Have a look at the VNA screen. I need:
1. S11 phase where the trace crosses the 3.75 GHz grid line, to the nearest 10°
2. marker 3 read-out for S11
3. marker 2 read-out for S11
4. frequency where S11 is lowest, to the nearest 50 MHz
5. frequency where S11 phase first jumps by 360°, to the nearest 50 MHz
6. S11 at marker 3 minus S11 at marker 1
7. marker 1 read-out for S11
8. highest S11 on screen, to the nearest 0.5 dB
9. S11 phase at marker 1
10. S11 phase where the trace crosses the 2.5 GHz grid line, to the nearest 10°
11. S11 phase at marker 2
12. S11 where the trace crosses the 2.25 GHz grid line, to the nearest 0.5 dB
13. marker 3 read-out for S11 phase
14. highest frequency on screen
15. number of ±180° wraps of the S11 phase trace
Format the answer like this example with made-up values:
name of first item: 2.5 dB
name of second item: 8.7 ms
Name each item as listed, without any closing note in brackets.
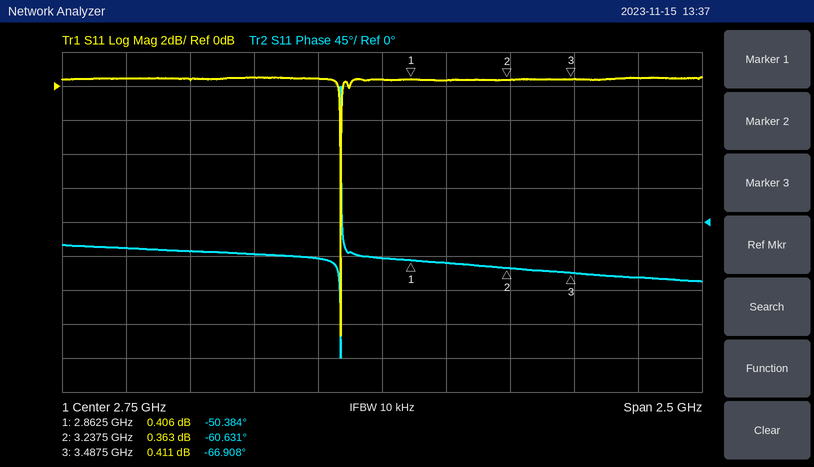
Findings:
S11 phase where the trace crosses the 3.75 GHz grid line, to the nearest 10°: -70°
marker 3 read-out for S11: 0.411 dB
marker 2 read-out for S11: 0.363 dB
frequency where S11 is lowest, to the nearest 50 MHz: 2.60 GHz
frequency where S11 phase first jumps by 360°, to the nearest 50 MHz: 2.60 GHz
S11 at marker 3 minus S11 at marker 1: 0.005 dB
marker 1 read-out for S11: 0.406 dB
highest S11 on screen, to the nearest 0.5 dB: 0.5 dB
S11 phase at marker 1: -50.384°
S11 phase where the trace crosses the 2.5 GHz grid line, to the nearest 10°: -50°
S11 phase at marker 2: -60.631°
S11 where the trace crosses the 2.25 GHz grid line, to the nearest 0.5 dB: 0.5 dB
marker 3 read-out for S11 phase: -66.908°
highest frequency on screen: 4 GHz
number of ±180° wraps of the S11 phase trace: 1
